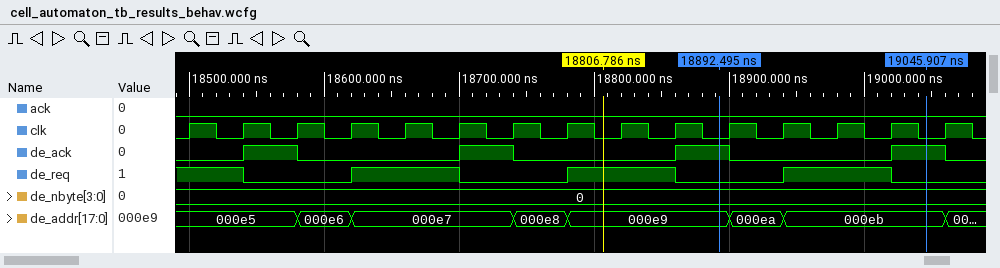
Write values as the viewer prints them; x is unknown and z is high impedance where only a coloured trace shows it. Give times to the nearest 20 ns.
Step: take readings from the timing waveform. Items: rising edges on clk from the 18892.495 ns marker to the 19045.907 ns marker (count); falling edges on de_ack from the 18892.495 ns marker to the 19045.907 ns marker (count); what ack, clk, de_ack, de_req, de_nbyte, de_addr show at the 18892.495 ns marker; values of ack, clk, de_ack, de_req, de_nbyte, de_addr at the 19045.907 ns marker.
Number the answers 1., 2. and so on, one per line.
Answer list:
1. 4
2. 1
3. ack=0, clk=0, de_ack=1, de_req=0, de_nbyte=0, de_addr=000e9
4. ack=0, clk=0, de_ack=1, de_req=0, de_nbyte=0, de_addr=000eb
